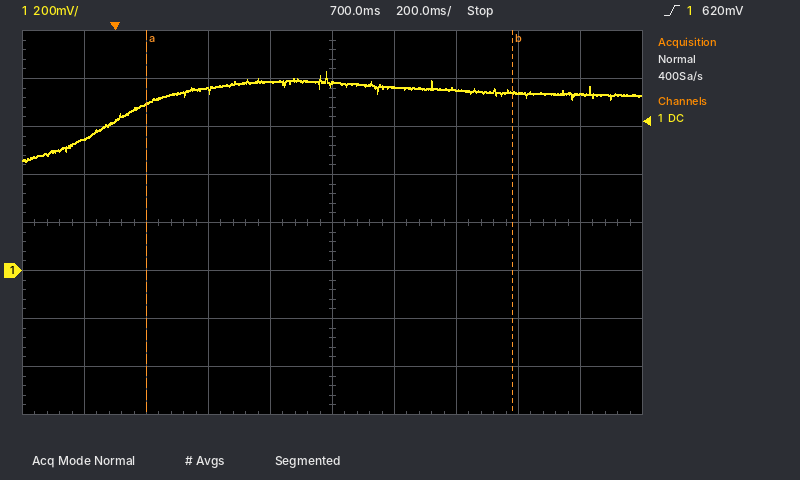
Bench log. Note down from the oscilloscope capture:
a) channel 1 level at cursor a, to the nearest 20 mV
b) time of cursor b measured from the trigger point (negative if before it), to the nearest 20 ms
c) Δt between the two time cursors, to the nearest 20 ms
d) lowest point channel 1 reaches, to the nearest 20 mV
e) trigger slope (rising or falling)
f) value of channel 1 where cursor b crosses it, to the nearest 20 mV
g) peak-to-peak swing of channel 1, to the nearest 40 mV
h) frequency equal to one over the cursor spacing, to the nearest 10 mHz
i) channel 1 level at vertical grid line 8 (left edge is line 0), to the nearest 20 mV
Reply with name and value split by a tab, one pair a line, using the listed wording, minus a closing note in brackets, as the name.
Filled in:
channel 1 level at cursor a, to the nearest 20 mV	700 mV
time of cursor b measured from the trigger point (negative if before it), to the nearest 20 ms	+1.28 s
Δt between the two time cursors, to the nearest 20 ms	1.18 s
lowest point channel 1 reaches, to the nearest 20 mV	460 mV
trigger slope	rising
value of channel 1 where cursor b crosses it, to the nearest 20 mV	740 mV
peak-to-peak swing of channel 1, to the nearest 40 mV	360 mV
frequency equal to one over the cursor spacing, to the nearest 10 mHz	850 mHz
channel 1 level at vertical grid line 8 (left edge is line 0), to the nearest 20 mV	740 mV
